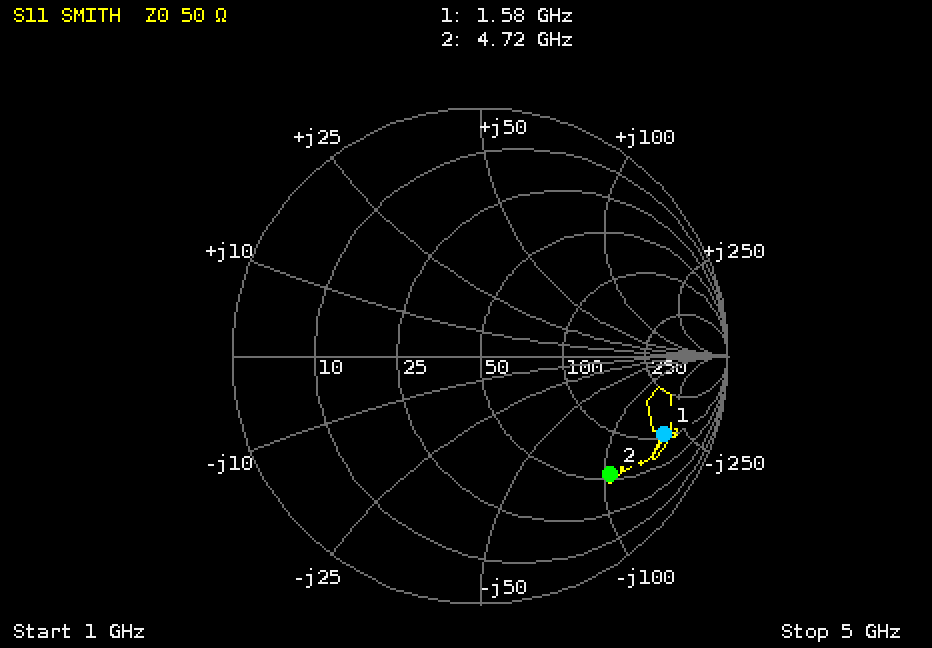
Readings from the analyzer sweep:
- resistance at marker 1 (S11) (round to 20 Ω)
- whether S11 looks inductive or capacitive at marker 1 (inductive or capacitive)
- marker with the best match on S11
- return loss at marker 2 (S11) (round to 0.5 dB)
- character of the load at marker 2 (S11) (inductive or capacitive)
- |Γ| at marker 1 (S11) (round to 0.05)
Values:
100 Ω
capacitive
marker 2
3.0 dB
capacitive
0.80
